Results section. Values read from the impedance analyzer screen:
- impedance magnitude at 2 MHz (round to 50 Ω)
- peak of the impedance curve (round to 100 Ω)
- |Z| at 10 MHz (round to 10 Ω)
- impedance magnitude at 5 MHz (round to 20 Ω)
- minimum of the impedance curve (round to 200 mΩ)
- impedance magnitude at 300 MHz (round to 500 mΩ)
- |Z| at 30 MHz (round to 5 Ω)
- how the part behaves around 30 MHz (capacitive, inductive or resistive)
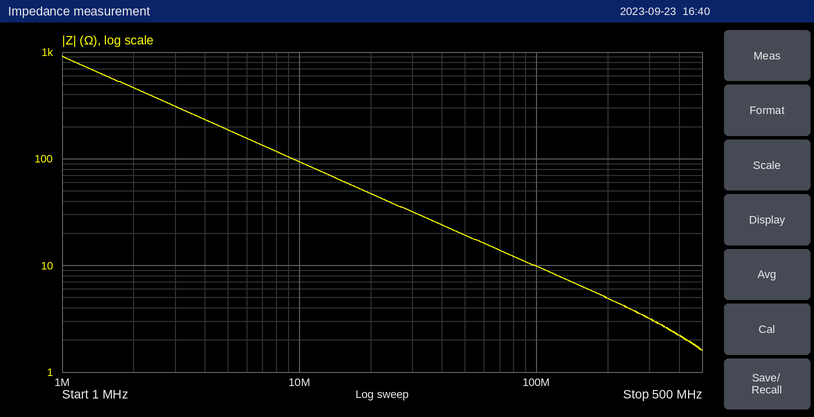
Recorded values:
450 Ω
900 Ω
90 Ω
180 Ω
1.6 Ω
3.0 Ω
30 Ω
capacitive
